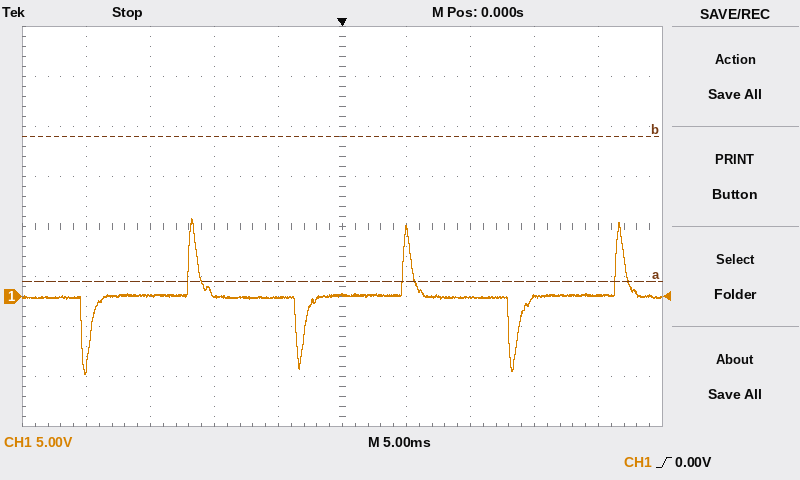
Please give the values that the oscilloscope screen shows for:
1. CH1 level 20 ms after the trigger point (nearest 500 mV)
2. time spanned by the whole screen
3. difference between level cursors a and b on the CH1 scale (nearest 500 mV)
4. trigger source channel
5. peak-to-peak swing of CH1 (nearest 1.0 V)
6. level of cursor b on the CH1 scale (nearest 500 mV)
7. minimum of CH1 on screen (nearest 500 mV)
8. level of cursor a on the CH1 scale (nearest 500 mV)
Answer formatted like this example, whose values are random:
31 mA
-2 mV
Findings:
0.0 V
50 ms
14.5 V
CH1
16.0 V
16.0 V
-8.0 V
1.5 V
